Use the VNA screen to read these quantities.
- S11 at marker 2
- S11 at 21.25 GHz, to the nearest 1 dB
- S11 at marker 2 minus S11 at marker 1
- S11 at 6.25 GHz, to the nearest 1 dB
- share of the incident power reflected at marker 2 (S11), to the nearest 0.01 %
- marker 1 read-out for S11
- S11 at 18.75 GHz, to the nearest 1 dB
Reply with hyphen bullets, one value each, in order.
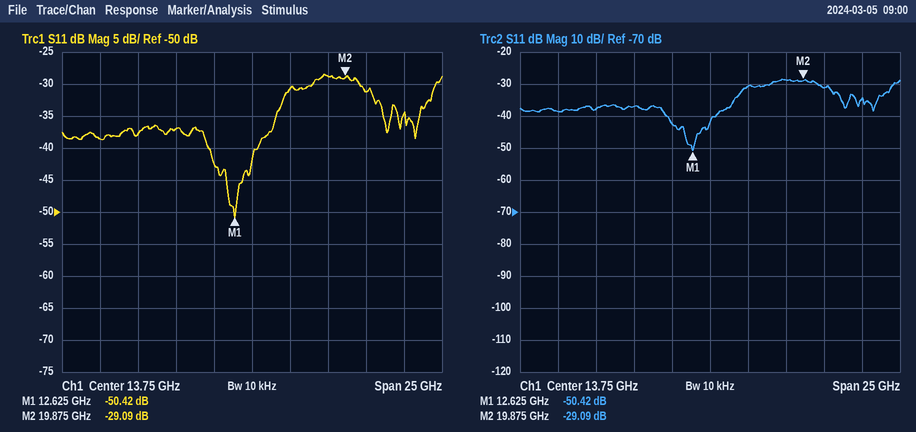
- -29.09 dB
- -31 dB
- 21.33 dB
- -38 dB
- 0.12 %
- -50.42 dB
- -29 dB
